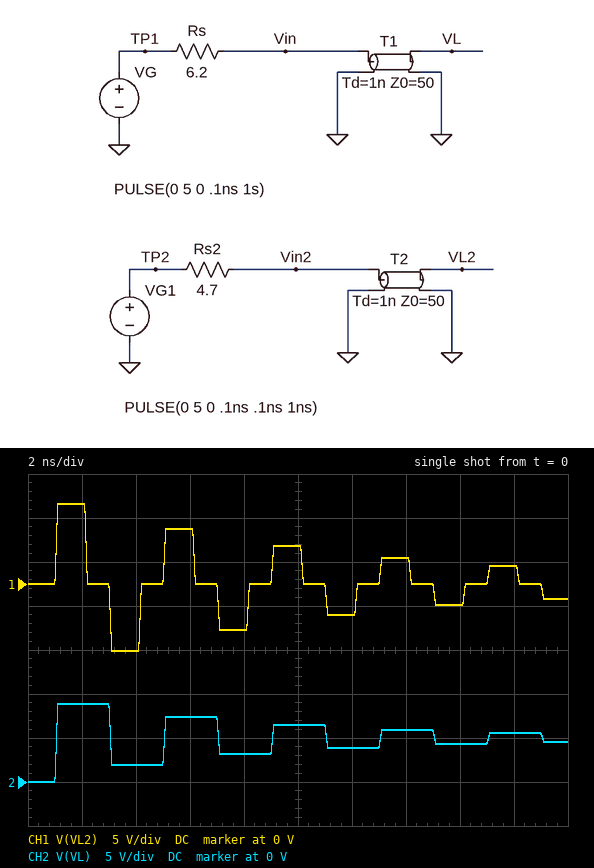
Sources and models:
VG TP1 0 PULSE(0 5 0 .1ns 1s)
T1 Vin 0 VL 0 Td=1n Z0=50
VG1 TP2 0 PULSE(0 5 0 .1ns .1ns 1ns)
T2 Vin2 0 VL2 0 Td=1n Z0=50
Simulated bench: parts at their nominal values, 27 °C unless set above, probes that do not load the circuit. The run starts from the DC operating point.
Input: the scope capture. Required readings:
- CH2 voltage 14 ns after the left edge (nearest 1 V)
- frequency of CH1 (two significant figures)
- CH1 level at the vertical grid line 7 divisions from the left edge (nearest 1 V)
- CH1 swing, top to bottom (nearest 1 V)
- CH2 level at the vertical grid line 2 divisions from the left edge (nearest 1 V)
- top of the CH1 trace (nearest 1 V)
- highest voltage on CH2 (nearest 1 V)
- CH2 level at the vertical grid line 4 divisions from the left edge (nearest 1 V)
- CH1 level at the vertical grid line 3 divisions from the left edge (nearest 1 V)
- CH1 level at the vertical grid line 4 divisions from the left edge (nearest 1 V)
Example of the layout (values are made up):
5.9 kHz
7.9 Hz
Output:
6 V
250 MHz
3 V
17 V
2 V
9 V
9 V
3 V
6 V
-5 V
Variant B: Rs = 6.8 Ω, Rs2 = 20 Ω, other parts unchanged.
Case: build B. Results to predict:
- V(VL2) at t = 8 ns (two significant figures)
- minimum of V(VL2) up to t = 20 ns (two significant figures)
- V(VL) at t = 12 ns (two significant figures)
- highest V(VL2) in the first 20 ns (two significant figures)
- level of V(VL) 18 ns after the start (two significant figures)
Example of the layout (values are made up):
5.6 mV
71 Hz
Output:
-560 mV
-3.1 V
4.0 V
7.1 V
5.4 V
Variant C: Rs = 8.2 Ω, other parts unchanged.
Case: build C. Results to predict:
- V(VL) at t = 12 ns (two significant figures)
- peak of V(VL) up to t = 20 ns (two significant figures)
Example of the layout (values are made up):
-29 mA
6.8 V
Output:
4.3 V
8.6 V
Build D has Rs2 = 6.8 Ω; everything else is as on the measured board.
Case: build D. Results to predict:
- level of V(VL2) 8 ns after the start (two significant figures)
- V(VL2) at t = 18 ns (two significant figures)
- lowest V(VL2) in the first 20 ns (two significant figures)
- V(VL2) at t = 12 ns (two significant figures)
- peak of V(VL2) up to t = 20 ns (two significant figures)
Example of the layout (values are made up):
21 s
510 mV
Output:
-3.9 V
990 mV
-6.7 V
-2.2 V
8.8 V
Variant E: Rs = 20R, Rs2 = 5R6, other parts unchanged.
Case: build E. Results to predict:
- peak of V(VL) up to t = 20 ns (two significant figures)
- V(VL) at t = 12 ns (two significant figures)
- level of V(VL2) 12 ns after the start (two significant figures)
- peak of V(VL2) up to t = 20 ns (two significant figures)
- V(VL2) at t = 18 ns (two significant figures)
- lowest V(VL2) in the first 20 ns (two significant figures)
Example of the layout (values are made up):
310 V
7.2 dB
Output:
7.1 V
5.0 V
-2.9 V
9.0 V
1.5 V
-7.2 V
